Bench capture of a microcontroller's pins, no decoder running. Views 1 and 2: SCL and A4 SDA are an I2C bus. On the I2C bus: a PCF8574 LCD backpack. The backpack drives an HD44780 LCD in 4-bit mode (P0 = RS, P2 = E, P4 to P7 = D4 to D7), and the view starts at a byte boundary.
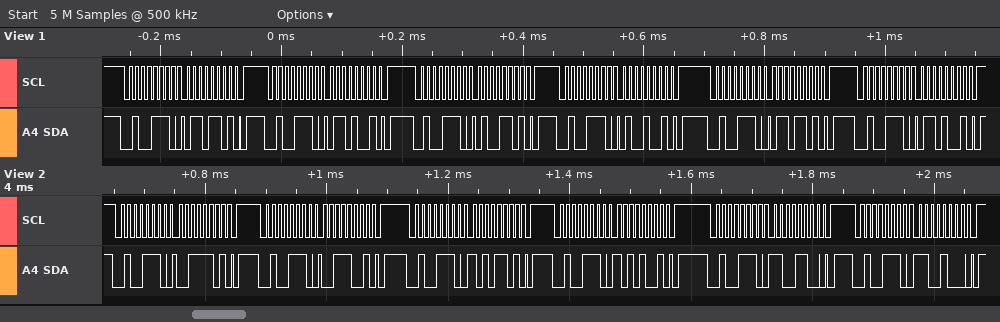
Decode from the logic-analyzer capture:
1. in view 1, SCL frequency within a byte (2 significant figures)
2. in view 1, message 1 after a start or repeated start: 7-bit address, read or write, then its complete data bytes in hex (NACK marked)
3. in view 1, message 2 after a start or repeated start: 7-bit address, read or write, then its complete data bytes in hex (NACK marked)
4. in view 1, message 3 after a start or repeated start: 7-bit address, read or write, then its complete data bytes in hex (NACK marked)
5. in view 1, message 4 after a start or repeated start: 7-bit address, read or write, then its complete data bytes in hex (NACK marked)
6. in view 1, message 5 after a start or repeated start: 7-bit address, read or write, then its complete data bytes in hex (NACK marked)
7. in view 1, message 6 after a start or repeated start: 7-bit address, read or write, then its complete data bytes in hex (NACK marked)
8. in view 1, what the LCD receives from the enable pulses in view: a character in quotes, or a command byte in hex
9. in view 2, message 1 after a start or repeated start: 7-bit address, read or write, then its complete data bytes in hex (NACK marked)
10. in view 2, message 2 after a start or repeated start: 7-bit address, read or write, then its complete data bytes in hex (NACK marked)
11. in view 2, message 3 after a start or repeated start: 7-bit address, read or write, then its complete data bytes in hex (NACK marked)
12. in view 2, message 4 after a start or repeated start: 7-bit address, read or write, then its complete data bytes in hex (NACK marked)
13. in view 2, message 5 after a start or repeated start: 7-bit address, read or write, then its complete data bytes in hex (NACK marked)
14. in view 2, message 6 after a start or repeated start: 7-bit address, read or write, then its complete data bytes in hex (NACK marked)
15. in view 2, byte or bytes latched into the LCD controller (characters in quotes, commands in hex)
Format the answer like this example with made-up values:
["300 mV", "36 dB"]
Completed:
["100 kHz", "0x27 write: 6D", "0x27 write: 69", "0x27 write: 4D", "0x27 write: 49", "0x27 write: 6D", "0x27 write: 69", "'d'", "0x27 write: 3D", "0x27 write: 39", "0x27 write: AD", "0x27 write: A9", "0x27 write: CC", "0x27 write: C8", "':'"]
